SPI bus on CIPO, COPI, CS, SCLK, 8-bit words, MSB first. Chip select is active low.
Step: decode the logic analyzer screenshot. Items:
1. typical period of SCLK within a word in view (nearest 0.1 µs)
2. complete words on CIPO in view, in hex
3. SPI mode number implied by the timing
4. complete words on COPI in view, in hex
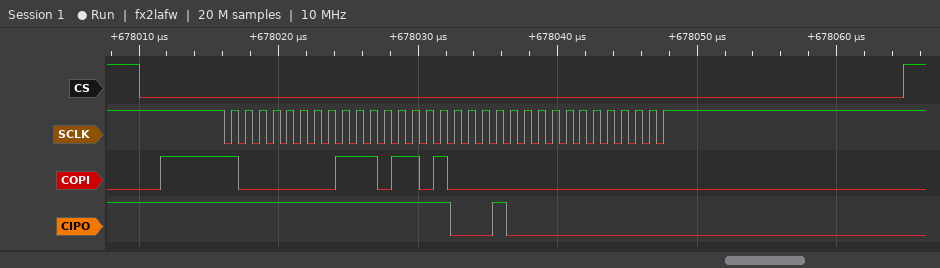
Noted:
1 µs
FF, FF, 10, 00
3
80, ED, 00, 00
